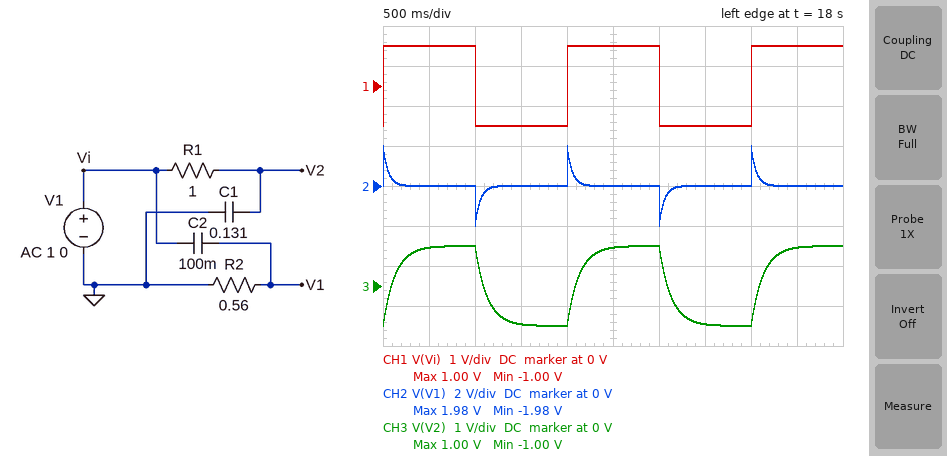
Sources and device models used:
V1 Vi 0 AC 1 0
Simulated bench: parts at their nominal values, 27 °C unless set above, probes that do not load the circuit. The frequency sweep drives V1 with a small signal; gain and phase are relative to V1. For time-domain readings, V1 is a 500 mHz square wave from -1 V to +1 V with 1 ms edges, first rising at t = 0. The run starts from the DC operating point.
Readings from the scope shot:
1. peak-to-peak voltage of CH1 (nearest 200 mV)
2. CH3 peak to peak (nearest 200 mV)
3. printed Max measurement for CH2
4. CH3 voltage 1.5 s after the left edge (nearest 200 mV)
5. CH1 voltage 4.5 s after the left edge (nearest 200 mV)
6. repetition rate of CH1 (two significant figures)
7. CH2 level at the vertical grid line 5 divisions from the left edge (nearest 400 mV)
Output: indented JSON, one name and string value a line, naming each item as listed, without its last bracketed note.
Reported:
{
  "peak-to-peak voltage of CH1": "2.0 V",
  "CH3 peak to peak": "2.0 V",
  "printed Max measurement for CH2": "1.98 V",
  "CH3 voltage 1.5 s after the left edge": "-1.0 V",
  "CH1 voltage 4.5 s after the left edge": "1.0 V",
  "repetition rate of CH1": "500 mHz",
  "CH2 level at the vertical grid line 5 divisions from the left edge": "0 V"
}
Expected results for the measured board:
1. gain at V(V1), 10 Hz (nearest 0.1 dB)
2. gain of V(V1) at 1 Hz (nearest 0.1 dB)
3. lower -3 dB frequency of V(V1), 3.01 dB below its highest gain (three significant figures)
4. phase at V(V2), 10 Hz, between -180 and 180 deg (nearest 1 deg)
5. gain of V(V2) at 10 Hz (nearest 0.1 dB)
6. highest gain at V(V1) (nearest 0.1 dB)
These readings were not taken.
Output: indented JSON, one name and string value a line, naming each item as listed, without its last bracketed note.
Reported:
{
  "gain at V(V1), 10 Hz": "-0.3 dB",
  "gain of V(V1) at 1 Hz": "-9.6 dB",
  "lower -3 dB frequency of V(V1), 3.01 dB below its highest gain": "2.84 Hz",
  "phase at V(V2), 10 Hz, between -180 and 180 deg": "-83 deg",
  "gain of V(V2) at 10 Hz": "-18.4 dB",
  "highest gain at V(V1)": "0 dB"
}
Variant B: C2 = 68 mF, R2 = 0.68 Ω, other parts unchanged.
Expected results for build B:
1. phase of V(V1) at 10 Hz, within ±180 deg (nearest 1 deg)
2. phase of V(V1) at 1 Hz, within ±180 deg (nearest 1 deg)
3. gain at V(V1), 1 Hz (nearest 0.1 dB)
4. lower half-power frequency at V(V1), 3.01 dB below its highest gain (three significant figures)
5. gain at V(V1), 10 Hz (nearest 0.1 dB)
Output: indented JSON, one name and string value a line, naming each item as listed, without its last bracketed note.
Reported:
{
  "phase of V(V1) at 10 Hz, within ±180 deg": "19 deg",
  "phase of V(V1) at 1 Hz, within ±180 deg": "74 deg",
  "gain at V(V1), 1 Hz": "-11.1 dB",
  "lower half-power frequency at V(V1), 3.01 dB below its highest gain": "3.44 Hz",
  "gain at V(V1), 10 Hz": "-0.5 dB"
}
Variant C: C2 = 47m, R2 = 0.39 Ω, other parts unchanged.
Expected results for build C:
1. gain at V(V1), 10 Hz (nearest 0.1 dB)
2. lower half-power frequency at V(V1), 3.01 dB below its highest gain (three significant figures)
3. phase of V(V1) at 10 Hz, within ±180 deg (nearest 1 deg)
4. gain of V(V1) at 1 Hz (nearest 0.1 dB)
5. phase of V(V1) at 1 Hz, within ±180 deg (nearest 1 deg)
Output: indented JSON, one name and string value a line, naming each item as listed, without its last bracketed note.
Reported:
{
  "gain at V(V1), 10 Hz": "-2.4 dB",
  "lower half-power frequency at V(V1), 3.01 dB below its highest gain": "8.68 Hz",
  "phase of V(V1) at 10 Hz, within ±180 deg": "41 deg",
  "gain of V(V1) at 1 Hz": "-18.8 dB",
  "phase of V(V1) at 1 Hz, within ±180 deg": "83 deg"
}
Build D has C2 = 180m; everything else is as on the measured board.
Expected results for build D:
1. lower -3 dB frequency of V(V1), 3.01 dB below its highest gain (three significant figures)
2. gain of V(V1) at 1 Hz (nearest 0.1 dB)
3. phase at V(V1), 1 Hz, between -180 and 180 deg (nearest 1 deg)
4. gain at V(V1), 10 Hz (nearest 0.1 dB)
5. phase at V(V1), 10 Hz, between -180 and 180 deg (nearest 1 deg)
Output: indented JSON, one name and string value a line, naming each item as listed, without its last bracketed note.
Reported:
{
  "lower -3 dB frequency of V(V1), 3.01 dB below its highest gain": "1.58 Hz",
  "gain of V(V1) at 1 Hz": "-5.4 dB",
  "phase at V(V1), 1 Hz, between -180 and 180 deg": "58 deg",
  "gain at V(V1), 10 Hz": "-0.1 dB",
  "phase at V(V1), 10 Hz, between -180 and 180 deg": "9 deg"
}
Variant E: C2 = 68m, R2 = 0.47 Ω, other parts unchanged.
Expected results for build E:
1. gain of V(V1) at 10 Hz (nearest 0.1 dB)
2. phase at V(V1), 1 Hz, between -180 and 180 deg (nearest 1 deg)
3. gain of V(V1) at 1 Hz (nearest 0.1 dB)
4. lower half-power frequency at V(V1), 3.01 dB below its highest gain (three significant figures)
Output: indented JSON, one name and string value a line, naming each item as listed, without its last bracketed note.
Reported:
{
  "gain of V(V1) at 10 Hz": "-1.0 dB",
  "phase at V(V1), 1 Hz, between -180 and 180 deg": "79 deg",
  "gain of V(V1) at 1 Hz": "-14.1 dB",
  "lower half-power frequency at V(V1), 3.01 dB below its highest gain": "4.98 Hz"
}
